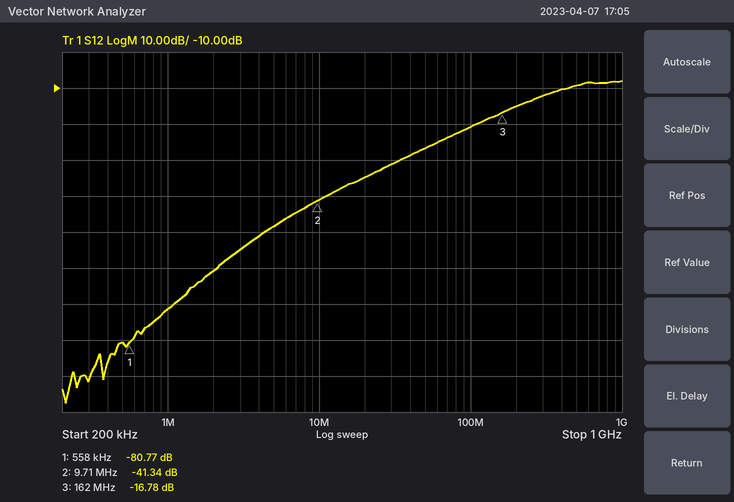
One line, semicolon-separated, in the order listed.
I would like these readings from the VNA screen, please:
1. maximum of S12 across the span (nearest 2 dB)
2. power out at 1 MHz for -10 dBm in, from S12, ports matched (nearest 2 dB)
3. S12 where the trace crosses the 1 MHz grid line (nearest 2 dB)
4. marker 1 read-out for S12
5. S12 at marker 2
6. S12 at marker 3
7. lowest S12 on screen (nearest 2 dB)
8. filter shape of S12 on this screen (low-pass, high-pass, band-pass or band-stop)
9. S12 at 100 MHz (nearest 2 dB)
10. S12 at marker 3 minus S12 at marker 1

-8 dB; -82 dBm; -72 dB; -80.77 dB; -41.34 dB; -16.78 dB; -98 dB; high-pass; -20 dB; 63.99 dB
